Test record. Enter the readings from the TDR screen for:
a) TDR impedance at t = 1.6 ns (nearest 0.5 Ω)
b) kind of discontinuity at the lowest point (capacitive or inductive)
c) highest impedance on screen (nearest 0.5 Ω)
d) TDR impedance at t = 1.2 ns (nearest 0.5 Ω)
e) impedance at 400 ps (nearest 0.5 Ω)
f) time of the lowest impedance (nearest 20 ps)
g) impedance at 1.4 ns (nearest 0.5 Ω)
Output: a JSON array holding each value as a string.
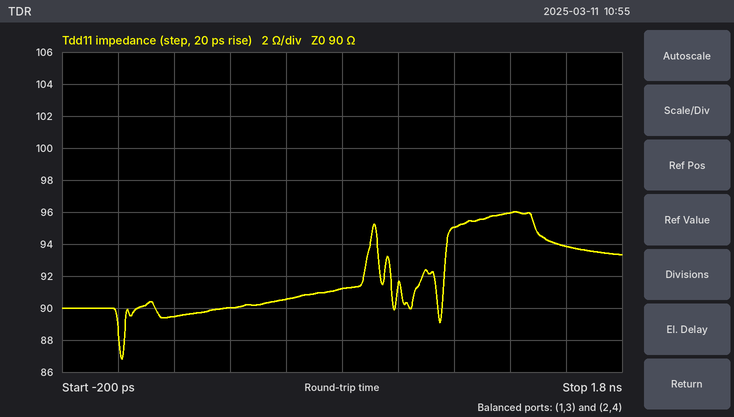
["94.0 Ω", "capacitive", "96.0 Ω", "95.0 Ω", "90.0 Ω", "20 ps", "96.0 Ω"]
